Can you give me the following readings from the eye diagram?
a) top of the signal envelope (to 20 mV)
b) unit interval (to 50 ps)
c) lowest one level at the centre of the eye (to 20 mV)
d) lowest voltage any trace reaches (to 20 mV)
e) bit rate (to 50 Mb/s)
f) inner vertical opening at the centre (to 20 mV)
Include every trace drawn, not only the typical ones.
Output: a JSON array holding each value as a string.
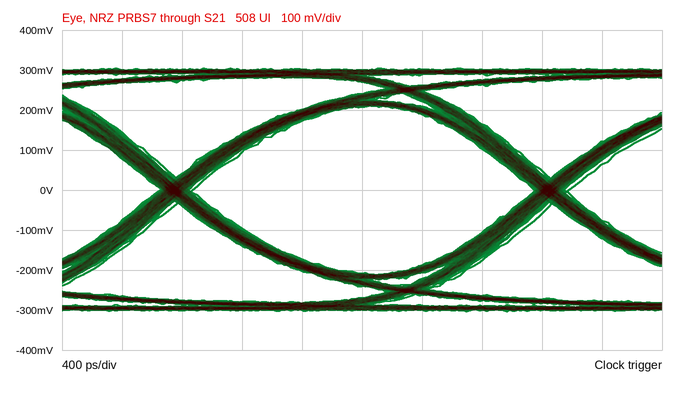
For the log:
["300 mV", "2.50 ns", "200 mV", "-300 mV", "400 Mb/s", "420 mV"]
